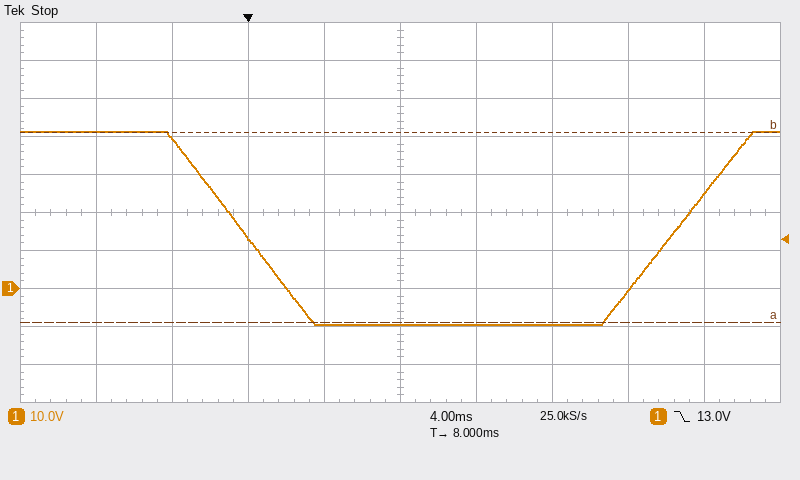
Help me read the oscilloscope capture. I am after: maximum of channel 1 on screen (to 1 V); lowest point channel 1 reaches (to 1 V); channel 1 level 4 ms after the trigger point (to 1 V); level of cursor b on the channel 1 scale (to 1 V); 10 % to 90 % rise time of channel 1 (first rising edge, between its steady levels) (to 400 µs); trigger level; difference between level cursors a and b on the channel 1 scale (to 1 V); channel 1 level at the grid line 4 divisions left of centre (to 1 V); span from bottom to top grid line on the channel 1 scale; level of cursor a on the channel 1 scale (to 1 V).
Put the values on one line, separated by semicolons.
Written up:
41 V; -9 V; -9 V; 41 V; 6.4 ms; 13.0 V; 50 V; 41 V; 100 V; -9 V
